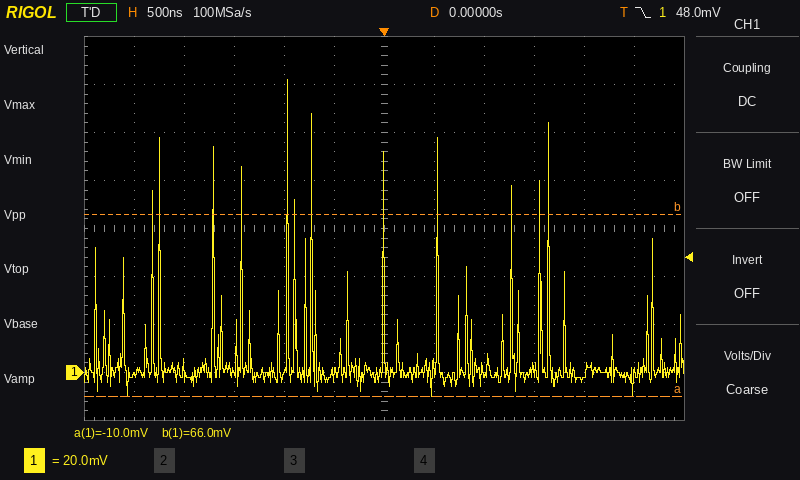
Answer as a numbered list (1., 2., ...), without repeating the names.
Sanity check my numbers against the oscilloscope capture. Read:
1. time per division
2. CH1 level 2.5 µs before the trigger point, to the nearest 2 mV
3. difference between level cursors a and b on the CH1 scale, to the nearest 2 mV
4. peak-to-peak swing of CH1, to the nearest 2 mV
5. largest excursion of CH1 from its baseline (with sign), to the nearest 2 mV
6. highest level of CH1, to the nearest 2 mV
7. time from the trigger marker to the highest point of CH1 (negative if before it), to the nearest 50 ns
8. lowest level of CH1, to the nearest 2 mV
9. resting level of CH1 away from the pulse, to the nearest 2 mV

1. 500 ns
2. 0 mV
3. 76 mV
4. 132 mV
5. +122 mV
6. 122 mV
7. -950 ns
8. -10 mV
9. 0 mV
